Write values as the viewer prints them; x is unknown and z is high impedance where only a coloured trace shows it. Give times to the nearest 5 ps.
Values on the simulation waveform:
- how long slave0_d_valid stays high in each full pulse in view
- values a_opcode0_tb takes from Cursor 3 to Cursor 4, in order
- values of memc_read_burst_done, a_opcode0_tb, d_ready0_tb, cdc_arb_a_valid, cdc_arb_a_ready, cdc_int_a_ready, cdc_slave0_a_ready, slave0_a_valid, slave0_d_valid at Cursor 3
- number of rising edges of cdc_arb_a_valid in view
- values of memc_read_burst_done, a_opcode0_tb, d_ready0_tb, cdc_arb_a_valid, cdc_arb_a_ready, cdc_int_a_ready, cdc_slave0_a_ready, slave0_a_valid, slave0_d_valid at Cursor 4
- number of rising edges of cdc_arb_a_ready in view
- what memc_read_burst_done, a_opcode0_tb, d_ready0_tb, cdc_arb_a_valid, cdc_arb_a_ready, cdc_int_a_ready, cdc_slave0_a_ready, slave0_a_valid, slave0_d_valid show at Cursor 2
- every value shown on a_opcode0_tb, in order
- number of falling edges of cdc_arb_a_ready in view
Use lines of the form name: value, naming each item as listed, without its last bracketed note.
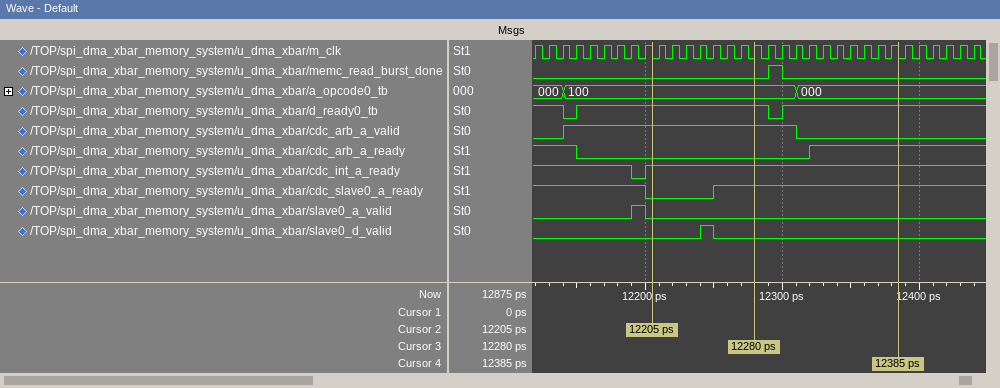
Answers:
how long slave0_d_valid stays high in each full pulse in view: 10 ps
values a_opcode0_tb takes from Cursor 3 to Cursor 4, in order: 100, 000
values of memc_read_burst_done, a_opcode0_tb, d_ready0_tb, cdc_arb_a_valid, cdc_arb_a_ready, cdc_int_a_ready, cdc_slave0_a_ready, slave0_a_valid, slave0_d_valid at Cursor 3: memc_read_burst_done=0, a_opcode0_tb=100, d_ready0_tb=1, cdc_arb_a_valid=1, cdc_arb_a_ready=0, cdc_int_a_ready=1, cdc_slave0_a_ready=1, slave0_a_valid=0, slave0_d_valid=0
number of rising edges of cdc_arb_a_valid in view: 1
values of memc_read_burst_done, a_opcode0_tb, d_ready0_tb, cdc_arb_a_valid, cdc_arb_a_ready, cdc_int_a_ready, cdc_slave0_a_ready, slave0_a_valid, slave0_d_valid at Cursor 4: memc_read_burst_done=0, a_opcode0_tb=000, d_ready0_tb=1, cdc_arb_a_valid=0, cdc_arb_a_ready=1, cdc_int_a_ready=1, cdc_slave0_a_ready=1, slave0_a_valid=0, slave0_d_valid=0
number of rising edges of cdc_arb_a_ready in view: 1
what memc_read_burst_done, a_opcode0_tb, d_ready0_tb, cdc_arb_a_valid, cdc_arb_a_ready, cdc_int_a_ready, cdc_slave0_a_ready, slave0_a_valid, slave0_d_valid show at Cursor 2: memc_read_burst_done=0, a_opcode0_tb=100, d_ready0_tb=1, cdc_arb_a_valid=1, cdc_arb_a_ready=0, cdc_int_a_ready=1, cdc_slave0_a_ready=0, slave0_a_valid=0, slave0_d_valid=0
every value shown on a_opcode0_tb, in order: 000, 100, 000
number of falling edges of cdc_arb_a_ready in view: 1
